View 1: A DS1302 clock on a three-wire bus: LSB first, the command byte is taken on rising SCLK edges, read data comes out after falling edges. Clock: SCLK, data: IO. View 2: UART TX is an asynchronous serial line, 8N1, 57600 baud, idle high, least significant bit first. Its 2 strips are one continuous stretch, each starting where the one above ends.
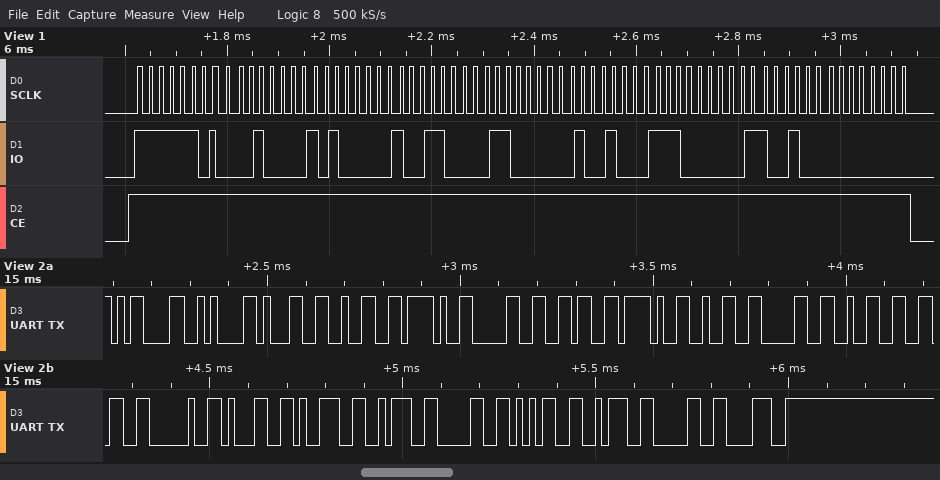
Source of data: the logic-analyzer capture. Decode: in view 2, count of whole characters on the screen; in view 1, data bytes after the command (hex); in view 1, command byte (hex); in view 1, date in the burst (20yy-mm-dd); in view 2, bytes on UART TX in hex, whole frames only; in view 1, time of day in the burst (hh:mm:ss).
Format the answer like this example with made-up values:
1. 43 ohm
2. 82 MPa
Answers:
1. 21
2. 08 05 19 06 12 07 26 00
3. 0xBF
4. 2026-12-06
5. 0D 0A 31 32 2F 30 36 2F 32 30 32 36 20 31 39 3A 30 35 3A 30 38
6. 19:05:08
